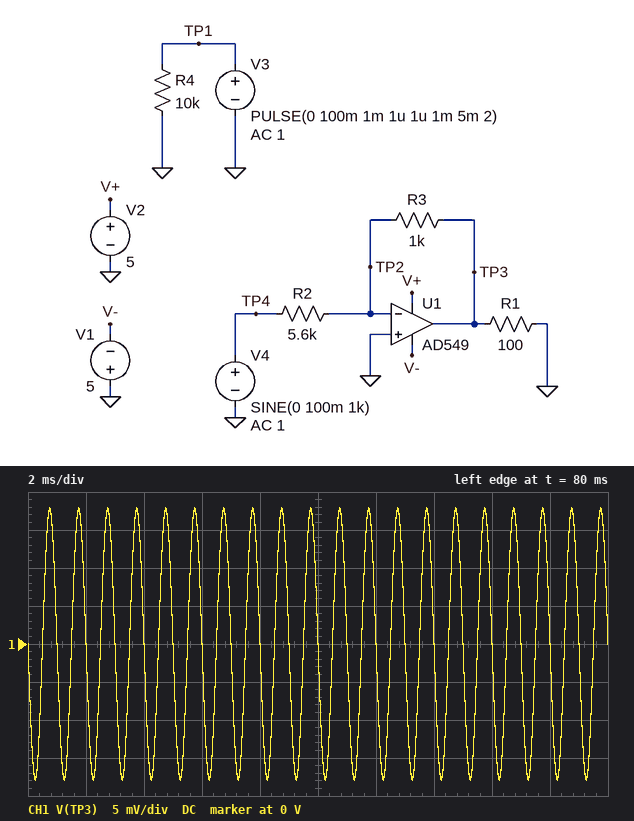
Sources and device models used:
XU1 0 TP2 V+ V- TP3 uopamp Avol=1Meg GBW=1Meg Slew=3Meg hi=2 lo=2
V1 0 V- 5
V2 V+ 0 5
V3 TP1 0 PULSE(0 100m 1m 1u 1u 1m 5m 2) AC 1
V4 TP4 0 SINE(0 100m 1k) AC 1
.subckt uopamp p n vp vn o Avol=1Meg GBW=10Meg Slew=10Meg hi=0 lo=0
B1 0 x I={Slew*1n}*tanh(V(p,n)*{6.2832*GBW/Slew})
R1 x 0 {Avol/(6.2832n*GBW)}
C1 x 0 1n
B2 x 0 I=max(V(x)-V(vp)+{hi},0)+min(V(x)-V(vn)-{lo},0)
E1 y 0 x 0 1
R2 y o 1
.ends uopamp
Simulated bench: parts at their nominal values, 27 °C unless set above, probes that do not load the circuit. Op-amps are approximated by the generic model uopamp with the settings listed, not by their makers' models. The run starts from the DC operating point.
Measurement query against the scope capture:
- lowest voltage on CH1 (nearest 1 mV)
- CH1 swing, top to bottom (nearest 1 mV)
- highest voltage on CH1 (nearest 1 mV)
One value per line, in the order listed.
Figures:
-18 mV
36 mV
18 mV
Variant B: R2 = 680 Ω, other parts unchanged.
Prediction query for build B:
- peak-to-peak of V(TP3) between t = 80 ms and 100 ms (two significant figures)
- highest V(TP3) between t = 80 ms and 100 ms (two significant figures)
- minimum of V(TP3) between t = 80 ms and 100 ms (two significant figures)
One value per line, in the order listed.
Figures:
290 mV
150 mV
-150 mV
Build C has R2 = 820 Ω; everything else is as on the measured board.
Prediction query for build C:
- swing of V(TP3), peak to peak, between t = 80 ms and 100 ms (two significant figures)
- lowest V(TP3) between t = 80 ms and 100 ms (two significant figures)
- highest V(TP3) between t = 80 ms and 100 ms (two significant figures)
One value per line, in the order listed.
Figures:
240 mV
-120 mV
120 mV
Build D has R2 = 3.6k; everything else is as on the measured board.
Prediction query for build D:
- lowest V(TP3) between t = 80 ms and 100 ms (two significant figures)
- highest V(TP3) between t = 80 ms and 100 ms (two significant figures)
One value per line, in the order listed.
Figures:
-28 mV
28 mV
